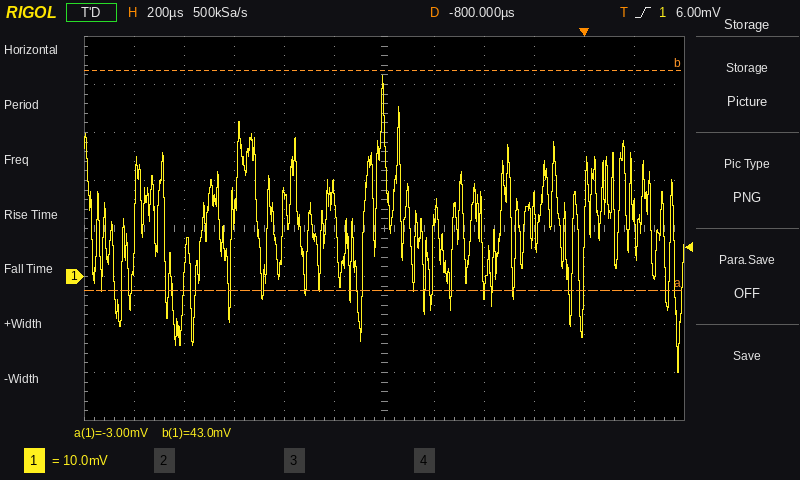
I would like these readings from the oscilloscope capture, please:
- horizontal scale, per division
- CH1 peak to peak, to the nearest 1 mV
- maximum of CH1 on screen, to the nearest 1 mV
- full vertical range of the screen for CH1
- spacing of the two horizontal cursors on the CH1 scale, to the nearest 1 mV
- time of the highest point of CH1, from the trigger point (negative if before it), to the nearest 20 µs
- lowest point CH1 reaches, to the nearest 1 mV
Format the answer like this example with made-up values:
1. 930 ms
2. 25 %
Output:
1. 200 µs
2. 62 mV
3. 42 mV
4. 80 mV
5. 46 mV
6. -800 µs
7. -20 mV
